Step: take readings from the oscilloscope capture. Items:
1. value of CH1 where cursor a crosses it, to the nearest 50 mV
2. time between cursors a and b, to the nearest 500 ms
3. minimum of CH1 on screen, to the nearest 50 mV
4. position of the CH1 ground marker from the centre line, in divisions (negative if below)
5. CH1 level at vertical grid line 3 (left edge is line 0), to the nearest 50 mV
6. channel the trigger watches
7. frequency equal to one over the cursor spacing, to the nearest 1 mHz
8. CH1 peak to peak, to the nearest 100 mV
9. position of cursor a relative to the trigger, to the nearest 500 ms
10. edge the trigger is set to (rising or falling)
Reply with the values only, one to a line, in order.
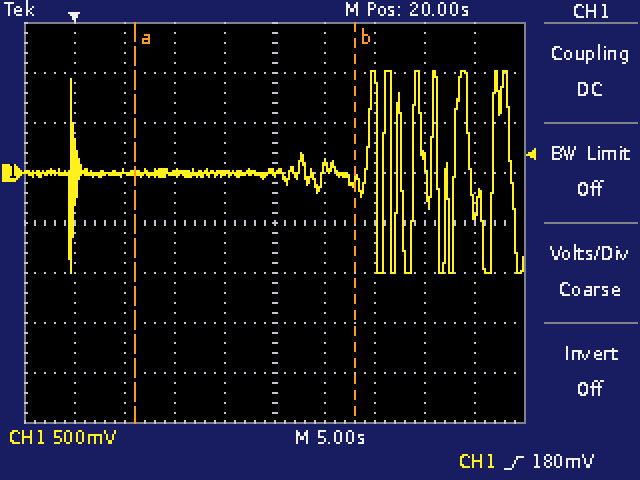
0 mV
22.0 s
-1.00 V
+1.0 div
0 mV
CH1
45 mHz
2.00 V
+6.0 s
rising
